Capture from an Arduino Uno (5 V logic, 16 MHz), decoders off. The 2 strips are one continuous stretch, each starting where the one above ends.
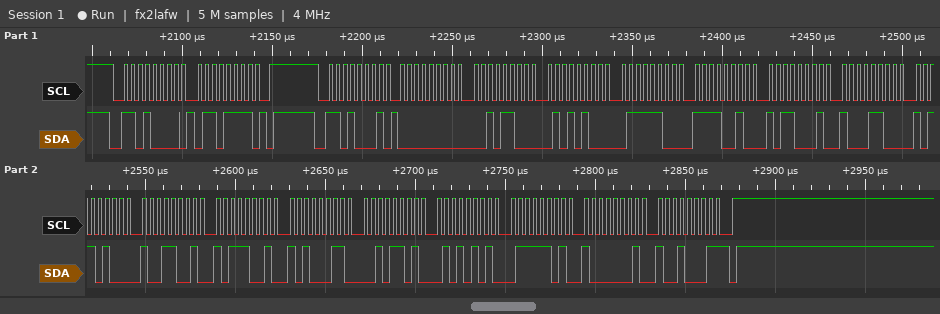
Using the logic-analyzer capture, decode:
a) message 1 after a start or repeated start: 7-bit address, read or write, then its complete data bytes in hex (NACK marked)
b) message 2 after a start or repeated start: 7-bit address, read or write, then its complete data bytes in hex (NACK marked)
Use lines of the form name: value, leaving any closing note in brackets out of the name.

message 1 after a start or repeated start: 7-bit address, read or write, then its complete data bytes in hex: 0x68 write: 6F
message 2 after a start or repeated start: 7-bit address, read or write, then its complete data bytes in hex: 0x68 read: 00 2C 54 7C F2 B1 8C B4 99 B9 A3 2D 55 7D 81 91 NACK
